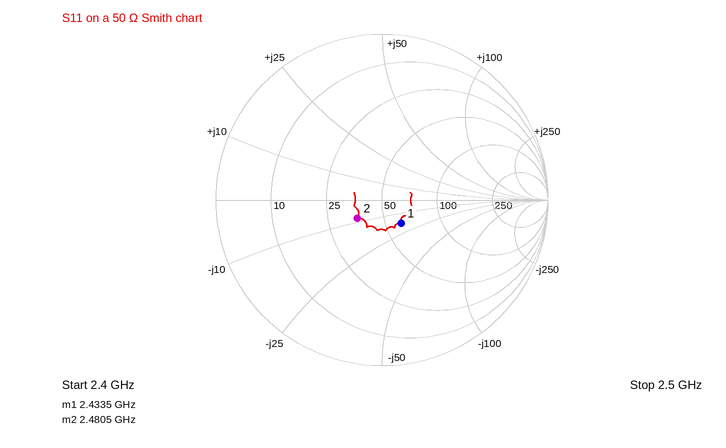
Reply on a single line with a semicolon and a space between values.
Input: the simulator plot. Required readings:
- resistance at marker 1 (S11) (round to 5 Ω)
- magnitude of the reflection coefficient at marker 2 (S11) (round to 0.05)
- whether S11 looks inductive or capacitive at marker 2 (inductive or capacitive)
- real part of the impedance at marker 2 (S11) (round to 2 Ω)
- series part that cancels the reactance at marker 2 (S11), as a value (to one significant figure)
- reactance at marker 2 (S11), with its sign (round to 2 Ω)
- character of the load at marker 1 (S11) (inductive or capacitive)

60 Ω; 0.20; capacitive; 36 Ω; 500 pH; -8 Ω; capacitive
